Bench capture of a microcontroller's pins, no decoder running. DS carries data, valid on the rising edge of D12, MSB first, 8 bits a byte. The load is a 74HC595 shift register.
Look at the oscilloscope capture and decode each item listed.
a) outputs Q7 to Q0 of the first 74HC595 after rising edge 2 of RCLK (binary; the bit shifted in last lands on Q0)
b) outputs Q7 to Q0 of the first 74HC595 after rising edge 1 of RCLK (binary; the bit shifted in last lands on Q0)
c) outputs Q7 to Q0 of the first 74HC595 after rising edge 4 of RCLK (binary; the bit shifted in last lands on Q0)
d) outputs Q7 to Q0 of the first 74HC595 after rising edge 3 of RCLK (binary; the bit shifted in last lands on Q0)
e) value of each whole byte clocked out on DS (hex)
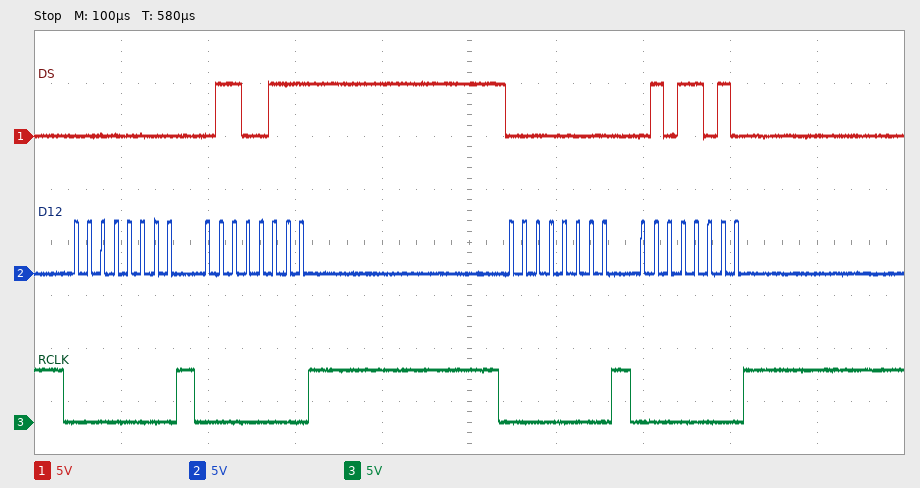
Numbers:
01100111
00000000
01011010
00000000
00 67 00 5A
